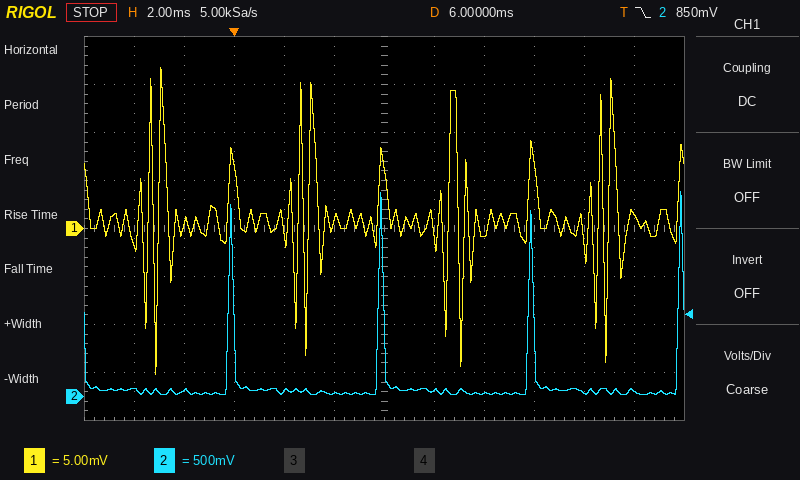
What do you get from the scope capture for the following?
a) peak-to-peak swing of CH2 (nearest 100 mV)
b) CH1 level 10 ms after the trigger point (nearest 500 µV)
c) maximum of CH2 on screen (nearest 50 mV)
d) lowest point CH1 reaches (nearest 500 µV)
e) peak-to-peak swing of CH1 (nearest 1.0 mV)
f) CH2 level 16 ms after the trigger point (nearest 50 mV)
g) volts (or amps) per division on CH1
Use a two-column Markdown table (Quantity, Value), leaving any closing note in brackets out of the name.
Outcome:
| Quantity | Value |
|---|---|
| peak-to-peak swing of CH2 | 2.10 V |
| CH1 level 10 ms after the trigger point | -500 µV |
| maximum of CH2 on screen | 2.15 V |
| lowest point CH1 reaches | -15.0 mV |
| peak-to-peak swing of CH1 | 32.0 mV |
| CH2 level 16 ms after the trigger point | 50 mV |
| volts (or amps) per division on CH1 | 5 mV |
